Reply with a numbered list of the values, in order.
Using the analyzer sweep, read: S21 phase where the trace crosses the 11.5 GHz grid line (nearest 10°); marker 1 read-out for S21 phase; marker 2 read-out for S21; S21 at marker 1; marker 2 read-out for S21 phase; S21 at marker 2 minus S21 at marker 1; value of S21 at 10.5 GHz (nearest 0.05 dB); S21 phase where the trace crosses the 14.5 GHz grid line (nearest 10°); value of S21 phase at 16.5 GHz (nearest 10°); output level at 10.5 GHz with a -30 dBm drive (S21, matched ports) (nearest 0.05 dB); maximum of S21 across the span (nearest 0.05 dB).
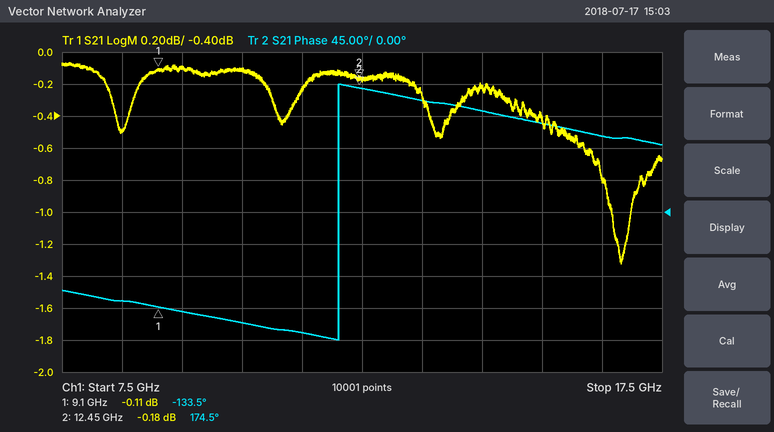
1. -170°
2. -133.5°
3. -0.18 dB
4. -0.11 dB
5. 174.5°
6. -0.07 dB
7. -0.10 dB
8. 140°
9. 110°
10. -30.10 dBm
11. -0.05 dB
